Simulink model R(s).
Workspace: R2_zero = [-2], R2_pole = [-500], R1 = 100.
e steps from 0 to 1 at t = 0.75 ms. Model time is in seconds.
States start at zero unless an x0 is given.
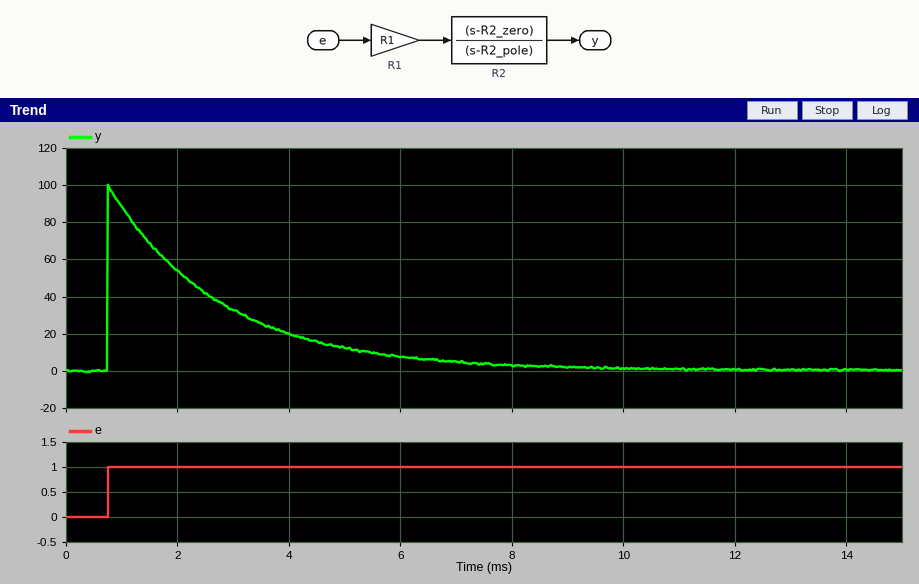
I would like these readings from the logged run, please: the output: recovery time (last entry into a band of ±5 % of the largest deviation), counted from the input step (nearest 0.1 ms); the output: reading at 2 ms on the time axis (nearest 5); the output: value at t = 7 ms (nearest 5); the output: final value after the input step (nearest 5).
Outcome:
6.0 ms
55
5
0
